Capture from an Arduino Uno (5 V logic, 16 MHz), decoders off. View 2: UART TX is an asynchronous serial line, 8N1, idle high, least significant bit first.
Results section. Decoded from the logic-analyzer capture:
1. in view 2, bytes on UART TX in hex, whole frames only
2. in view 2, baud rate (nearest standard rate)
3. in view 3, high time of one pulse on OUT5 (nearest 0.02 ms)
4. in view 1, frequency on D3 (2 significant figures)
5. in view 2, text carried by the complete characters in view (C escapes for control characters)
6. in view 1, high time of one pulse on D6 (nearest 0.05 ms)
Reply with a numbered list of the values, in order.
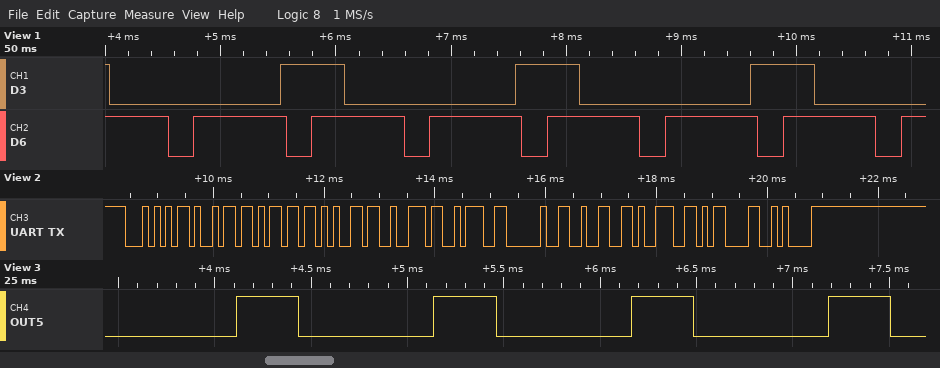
1. 0x54 0x69 0x6D 0x65 0x72 0x3A 0x20 0x32 0x39 0x0D 0x0A
2. 9600 baud
3. 0.32 ms
4. 490 Hz
5. "Timer: 29\r\n"
6. 0.80 ms
